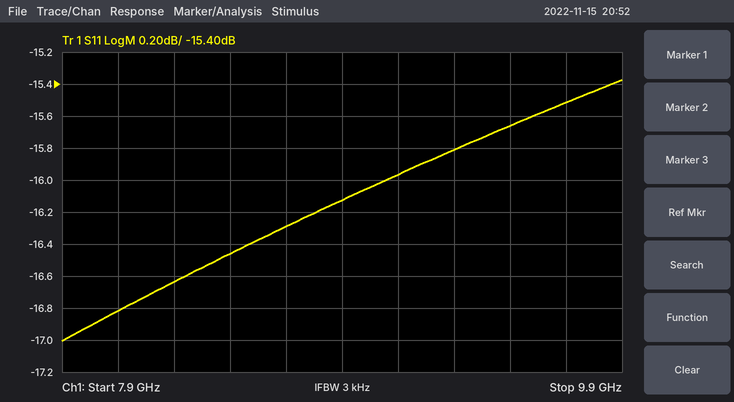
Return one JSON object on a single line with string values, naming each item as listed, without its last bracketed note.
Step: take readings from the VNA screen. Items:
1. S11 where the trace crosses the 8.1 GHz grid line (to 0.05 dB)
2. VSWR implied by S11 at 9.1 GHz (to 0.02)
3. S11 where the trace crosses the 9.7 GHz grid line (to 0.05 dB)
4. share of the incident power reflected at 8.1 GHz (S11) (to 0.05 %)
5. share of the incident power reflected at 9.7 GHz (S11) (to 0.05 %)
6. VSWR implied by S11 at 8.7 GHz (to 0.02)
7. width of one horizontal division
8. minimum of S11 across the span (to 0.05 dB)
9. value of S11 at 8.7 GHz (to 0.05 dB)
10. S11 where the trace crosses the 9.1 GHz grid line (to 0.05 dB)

{"S11 where the trace crosses the 8.1 GHz grid line": "-16.80 dB", "VSWR implied by S11 at 9.1 GHz": "1.38", "S11 where the trace crosses the 9.7 GHz grid line": "-15.50 dB", "share of the incident power reflected at 8.1 GHz (S11)": "2.10 %", "share of the incident power reflected at 9.7 GHz (S11)": "2.80 %", "VSWR implied by S11 at 8.7 GHz": "1.36", "width of one horizontal division": "200 MHz", "minimum of S11 across the span": "-17.00 dB", "value of S11 at 8.7 GHz": "-16.30 dB", "S11 where the trace crosses the 9.1 GHz grid line": "-15.95 dB"}
